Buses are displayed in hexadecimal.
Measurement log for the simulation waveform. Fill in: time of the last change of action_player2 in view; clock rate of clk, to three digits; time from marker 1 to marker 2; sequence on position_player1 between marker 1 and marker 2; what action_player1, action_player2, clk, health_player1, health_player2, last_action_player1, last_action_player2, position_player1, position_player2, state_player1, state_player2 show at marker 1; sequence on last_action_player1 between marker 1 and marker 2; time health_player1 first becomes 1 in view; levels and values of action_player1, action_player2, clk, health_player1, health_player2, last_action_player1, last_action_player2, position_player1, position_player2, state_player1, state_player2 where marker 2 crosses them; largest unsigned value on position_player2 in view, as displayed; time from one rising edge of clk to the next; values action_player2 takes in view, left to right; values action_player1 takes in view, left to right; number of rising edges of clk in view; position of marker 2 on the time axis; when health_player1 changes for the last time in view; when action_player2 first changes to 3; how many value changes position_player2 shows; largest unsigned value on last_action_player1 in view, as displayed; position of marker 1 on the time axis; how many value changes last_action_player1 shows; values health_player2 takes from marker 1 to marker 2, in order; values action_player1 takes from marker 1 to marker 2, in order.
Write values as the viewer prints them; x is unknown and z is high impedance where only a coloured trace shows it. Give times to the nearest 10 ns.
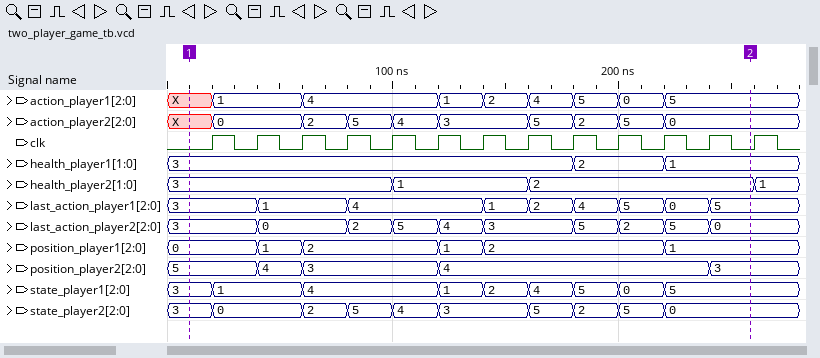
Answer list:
220 ns
50.0 MHz
250 ns
0, 1, 2, 1, 2, 1
action_player1=X, action_player2=X, clk=0, health_player1=3, health_player2=3, last_action_player1=3, last_action_player2=3, position_player1=0, position_player2=5, state_player1=3, state_player2=3
3, 1, 4, 1, 2, 4, 5, 0, 5
220 ns
action_player1=5, action_player2=0, clk=0, health_player1=1, health_player2=2, last_action_player1=5, last_action_player2=0, position_player1=1, position_player2=3, state_player1=5, state_player2=0
5
20 ns
X, 0, 2, 5, 4, 3, 5, 2, 5, 0
X, 1, 4, 1, 2, 4, 5, 0, 5
13
260 ns
220 ns
120 ns
4
5
10 ns
8
3, 1, 2
X, 1, 4, 1, 2, 4, 5, 0, 5
